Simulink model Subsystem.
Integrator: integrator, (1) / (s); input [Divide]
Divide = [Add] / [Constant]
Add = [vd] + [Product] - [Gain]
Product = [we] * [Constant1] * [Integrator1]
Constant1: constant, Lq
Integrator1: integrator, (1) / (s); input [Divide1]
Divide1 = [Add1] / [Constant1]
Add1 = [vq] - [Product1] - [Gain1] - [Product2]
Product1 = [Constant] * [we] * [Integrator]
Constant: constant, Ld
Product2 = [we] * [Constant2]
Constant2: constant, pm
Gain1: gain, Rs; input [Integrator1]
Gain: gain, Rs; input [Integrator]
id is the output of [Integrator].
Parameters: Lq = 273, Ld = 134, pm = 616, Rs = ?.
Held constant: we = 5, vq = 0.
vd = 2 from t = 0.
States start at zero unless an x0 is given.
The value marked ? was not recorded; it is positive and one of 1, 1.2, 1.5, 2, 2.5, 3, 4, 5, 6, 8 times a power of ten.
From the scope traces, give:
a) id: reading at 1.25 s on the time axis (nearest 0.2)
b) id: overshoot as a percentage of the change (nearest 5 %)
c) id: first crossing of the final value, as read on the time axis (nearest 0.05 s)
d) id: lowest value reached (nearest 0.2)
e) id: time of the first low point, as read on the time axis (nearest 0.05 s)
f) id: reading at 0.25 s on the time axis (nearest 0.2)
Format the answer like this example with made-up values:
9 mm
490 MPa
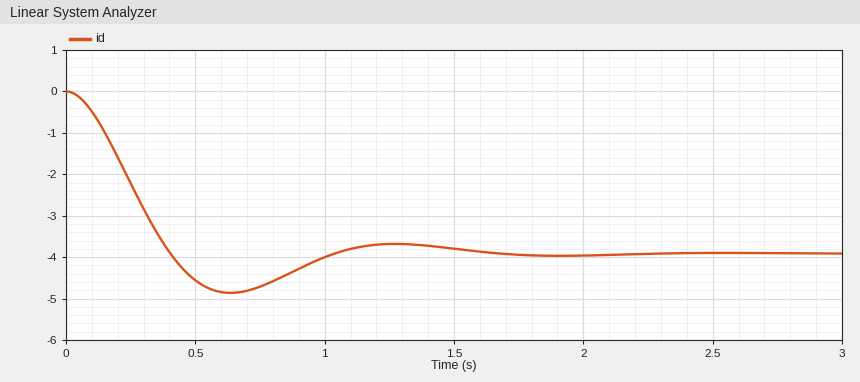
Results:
-3.6
25 %
0.40 s
-4.8
0.65 s
-2.2
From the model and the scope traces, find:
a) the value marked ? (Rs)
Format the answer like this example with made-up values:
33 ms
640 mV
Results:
400
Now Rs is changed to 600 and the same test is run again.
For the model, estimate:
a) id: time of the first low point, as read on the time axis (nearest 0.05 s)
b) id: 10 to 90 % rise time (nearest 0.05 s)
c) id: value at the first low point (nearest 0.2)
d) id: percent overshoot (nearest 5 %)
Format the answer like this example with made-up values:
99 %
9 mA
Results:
0.65 s
0.30 s
-3.6
10 %
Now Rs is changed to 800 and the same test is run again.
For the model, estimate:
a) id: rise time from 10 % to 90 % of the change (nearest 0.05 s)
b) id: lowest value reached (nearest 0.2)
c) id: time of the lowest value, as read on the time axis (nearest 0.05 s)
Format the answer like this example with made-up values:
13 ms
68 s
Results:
0.30 s
-2.8
0.65 s
